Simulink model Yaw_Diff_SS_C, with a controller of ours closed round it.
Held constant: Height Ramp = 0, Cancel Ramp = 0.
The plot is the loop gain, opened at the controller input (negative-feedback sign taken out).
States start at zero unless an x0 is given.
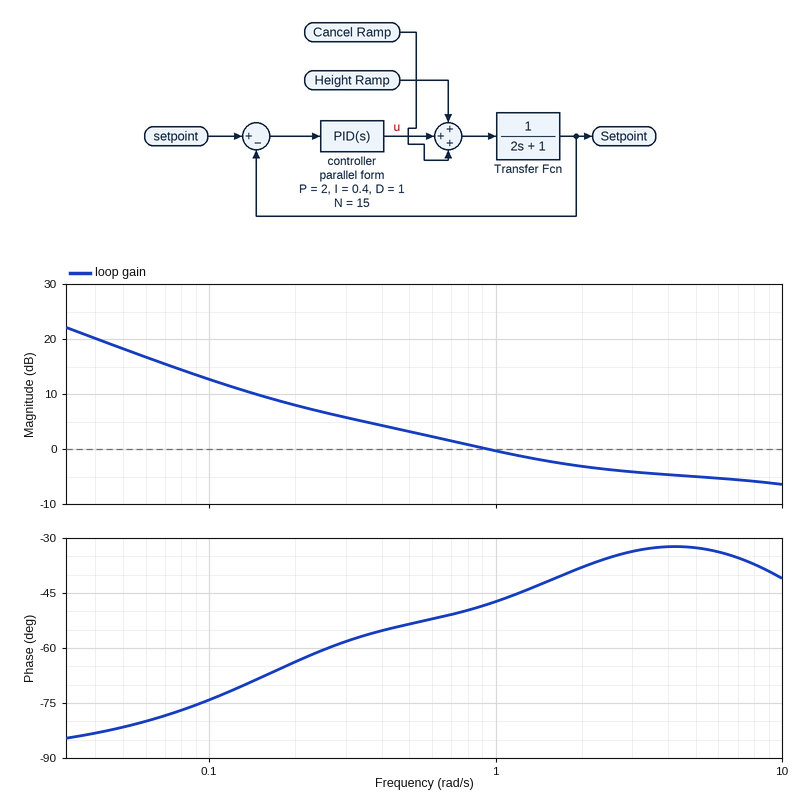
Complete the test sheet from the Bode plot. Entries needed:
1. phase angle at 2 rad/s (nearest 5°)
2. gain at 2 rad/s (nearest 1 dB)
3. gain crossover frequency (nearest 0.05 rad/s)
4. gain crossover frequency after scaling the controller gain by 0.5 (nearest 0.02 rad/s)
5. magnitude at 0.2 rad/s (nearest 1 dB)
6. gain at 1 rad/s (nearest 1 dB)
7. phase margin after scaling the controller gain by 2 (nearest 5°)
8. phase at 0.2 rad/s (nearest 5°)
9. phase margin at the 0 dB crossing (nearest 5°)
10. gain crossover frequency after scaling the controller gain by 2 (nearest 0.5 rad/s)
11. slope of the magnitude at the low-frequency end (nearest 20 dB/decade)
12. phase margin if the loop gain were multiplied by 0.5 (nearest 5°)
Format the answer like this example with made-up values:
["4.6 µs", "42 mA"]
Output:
["-40°", "-3 dB", "0.95 rad/s", "0.28 rad/s", "8 dB", "0 dB", "140°", "-65°", "130°", "8.5 rad/s", "-20 dB/decade", "120°"]
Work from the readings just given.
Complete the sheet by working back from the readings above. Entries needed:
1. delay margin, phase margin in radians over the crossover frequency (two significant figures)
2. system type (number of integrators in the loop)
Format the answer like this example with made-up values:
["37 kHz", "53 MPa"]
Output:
["2.4 s", "1"]
